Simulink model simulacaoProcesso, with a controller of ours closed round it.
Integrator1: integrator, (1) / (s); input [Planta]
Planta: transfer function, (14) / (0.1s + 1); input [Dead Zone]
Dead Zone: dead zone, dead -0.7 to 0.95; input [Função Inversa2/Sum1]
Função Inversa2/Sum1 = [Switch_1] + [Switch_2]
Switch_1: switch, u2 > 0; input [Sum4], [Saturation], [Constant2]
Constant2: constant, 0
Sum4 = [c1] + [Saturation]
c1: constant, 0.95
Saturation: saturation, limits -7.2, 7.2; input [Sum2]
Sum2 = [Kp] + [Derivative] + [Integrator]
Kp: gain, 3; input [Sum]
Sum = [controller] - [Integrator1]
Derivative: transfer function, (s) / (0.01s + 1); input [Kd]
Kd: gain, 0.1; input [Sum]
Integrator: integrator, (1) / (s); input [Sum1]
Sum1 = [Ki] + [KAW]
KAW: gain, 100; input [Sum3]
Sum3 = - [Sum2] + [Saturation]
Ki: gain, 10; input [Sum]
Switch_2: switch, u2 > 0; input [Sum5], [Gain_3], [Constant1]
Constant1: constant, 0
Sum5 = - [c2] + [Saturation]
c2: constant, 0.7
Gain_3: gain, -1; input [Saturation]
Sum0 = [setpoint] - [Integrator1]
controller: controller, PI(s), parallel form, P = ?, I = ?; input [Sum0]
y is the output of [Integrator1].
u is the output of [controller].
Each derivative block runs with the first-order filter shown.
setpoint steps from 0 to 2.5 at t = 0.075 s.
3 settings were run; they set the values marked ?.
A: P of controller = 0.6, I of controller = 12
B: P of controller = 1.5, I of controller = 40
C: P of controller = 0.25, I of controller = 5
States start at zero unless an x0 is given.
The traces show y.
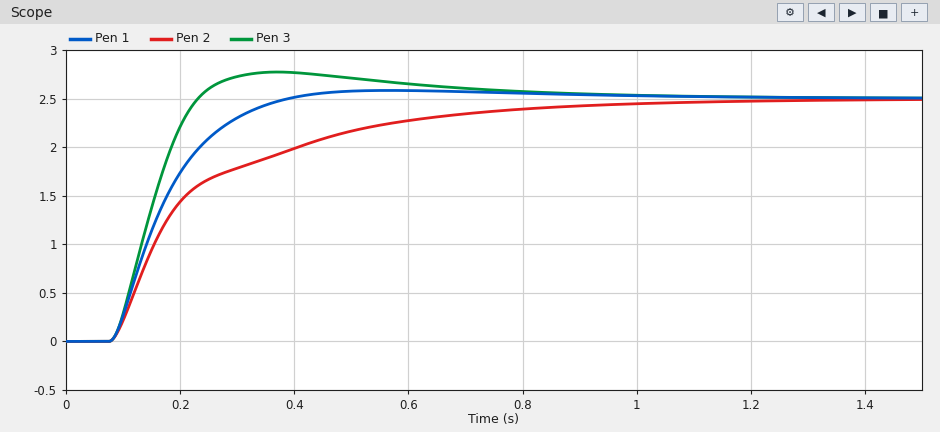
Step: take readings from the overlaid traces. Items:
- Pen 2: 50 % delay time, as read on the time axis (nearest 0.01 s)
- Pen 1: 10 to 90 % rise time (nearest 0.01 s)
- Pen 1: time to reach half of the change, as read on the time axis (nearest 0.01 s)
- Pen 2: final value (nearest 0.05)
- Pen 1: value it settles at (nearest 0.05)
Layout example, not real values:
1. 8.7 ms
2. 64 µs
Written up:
1. 0.18 s
2. 0.19 s
3. 0.16 s
4. 2.50
5. 2.50
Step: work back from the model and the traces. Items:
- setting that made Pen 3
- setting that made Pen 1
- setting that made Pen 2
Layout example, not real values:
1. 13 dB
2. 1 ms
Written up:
1. B
2. A
3. C
